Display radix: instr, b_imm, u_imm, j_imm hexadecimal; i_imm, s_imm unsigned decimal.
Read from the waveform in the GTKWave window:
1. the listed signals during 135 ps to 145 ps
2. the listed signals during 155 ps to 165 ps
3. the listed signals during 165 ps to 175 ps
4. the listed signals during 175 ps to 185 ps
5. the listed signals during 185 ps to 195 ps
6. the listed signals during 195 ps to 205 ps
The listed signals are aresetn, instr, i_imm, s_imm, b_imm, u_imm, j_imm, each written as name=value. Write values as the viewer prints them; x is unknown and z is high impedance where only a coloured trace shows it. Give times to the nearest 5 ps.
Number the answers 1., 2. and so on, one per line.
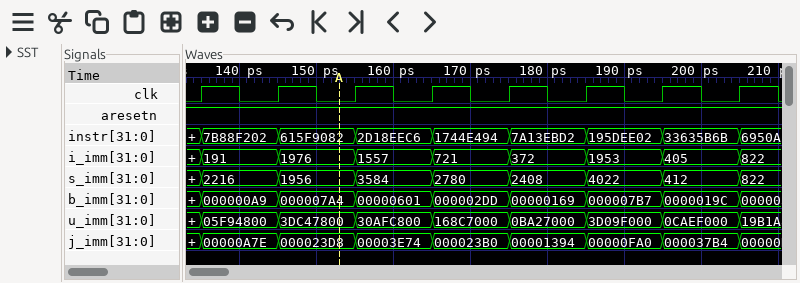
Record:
1. aresetn=1, instr=7B88F202, i_imm=191, s_imm=2216, b_imm=000000A9, u_imm=05F94800, j_imm=00000A7E
2. aresetn=1, instr=2D18EEC6, i_imm=1557, s_imm=3584, b_imm=00000601, u_imm=30AFC800, j_imm=00003E74
3. aresetn=1, instr=1744E494, i_imm=721, s_imm=2780, b_imm=000002DD, u_imm=168C7000, j_imm=000023B0
4. aresetn=1, instr=7A13EBD2, i_imm=372, s_imm=2408, b_imm=00000169, u_imm=0BA27000, j_imm=00001394
5. aresetn=1, instr=195DEE02, i_imm=1953, s_imm=4022, b_imm=000007B7, u_imm=3D09F000, j_imm=00000FA0
6. aresetn=1, instr=33635B6B, i_imm=405, s_imm=412, b_imm=0000019C, u_imm=0CAEF000, j_imm=000037B4
